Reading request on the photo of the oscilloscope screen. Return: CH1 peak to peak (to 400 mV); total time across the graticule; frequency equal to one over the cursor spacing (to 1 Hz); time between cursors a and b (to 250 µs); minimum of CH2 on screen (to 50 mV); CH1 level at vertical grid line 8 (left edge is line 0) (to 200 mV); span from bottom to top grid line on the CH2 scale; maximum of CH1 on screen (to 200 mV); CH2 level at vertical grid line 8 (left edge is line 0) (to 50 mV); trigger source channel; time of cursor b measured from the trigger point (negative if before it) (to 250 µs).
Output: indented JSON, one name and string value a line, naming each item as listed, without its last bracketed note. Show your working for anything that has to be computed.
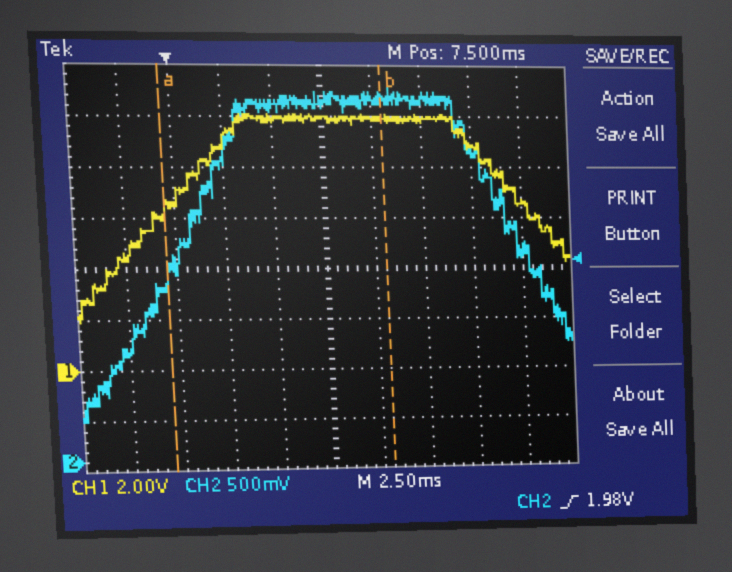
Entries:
{
  "CH1 peak to peak": "8.0 V",
  "total time across the graticule": "25 ms",
  "frequency equal to one over the cursor spacing": "1 / 11.00 ms ≈ 91 Hz",
  "time between cursors a and b": "11.00 ms",
  "minimum of CH2 on screen": "400 mV",
  "CH1 level at vertical grid line 8 (left edge is line 0)": "8.8 V",
  "span from bottom to top grid line on the CH2 scale": "4 V",
  "maximum of CH1 on screen": "10.0 V",
  "CH2 level at vertical grid line 8 (left edge is line 0)": "3.05 V",
  "trigger source channel": "CH2",
  "time of cursor b measured from the trigger point (negative if before it)": "+10.50 ms"
}
